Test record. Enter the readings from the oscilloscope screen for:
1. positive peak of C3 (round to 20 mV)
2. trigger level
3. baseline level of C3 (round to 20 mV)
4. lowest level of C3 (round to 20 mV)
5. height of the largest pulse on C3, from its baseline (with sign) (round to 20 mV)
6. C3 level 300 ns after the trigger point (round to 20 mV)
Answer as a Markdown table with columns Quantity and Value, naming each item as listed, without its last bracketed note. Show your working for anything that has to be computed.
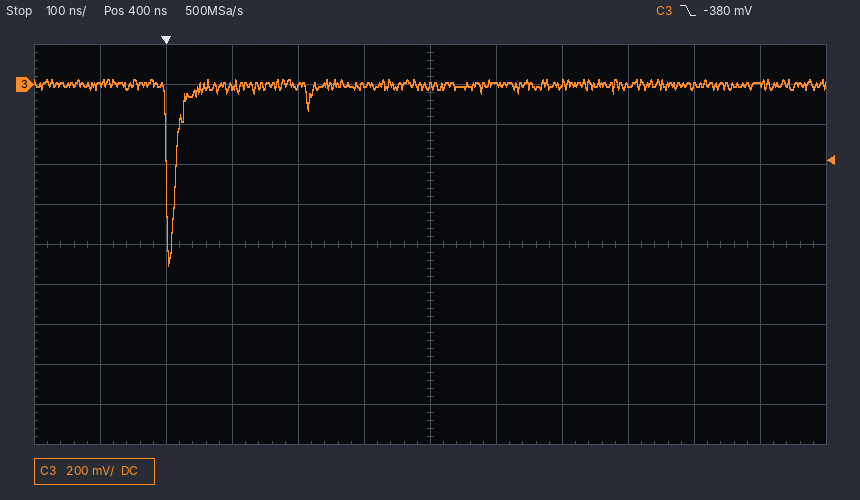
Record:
| Quantity | Value |
|---|---|
| positive peak of C3 | 20 mV |
| trigger level | -380 mV |
| baseline level of C3 | 0 mV |
| lowest level of C3 | -900 mV |
| height of the largest pulse on C3, from its baseline (with sign) | -900 mV − (0 mV) = -900 mV |
| C3 level 300 ns after the trigger point | 0 mV |
